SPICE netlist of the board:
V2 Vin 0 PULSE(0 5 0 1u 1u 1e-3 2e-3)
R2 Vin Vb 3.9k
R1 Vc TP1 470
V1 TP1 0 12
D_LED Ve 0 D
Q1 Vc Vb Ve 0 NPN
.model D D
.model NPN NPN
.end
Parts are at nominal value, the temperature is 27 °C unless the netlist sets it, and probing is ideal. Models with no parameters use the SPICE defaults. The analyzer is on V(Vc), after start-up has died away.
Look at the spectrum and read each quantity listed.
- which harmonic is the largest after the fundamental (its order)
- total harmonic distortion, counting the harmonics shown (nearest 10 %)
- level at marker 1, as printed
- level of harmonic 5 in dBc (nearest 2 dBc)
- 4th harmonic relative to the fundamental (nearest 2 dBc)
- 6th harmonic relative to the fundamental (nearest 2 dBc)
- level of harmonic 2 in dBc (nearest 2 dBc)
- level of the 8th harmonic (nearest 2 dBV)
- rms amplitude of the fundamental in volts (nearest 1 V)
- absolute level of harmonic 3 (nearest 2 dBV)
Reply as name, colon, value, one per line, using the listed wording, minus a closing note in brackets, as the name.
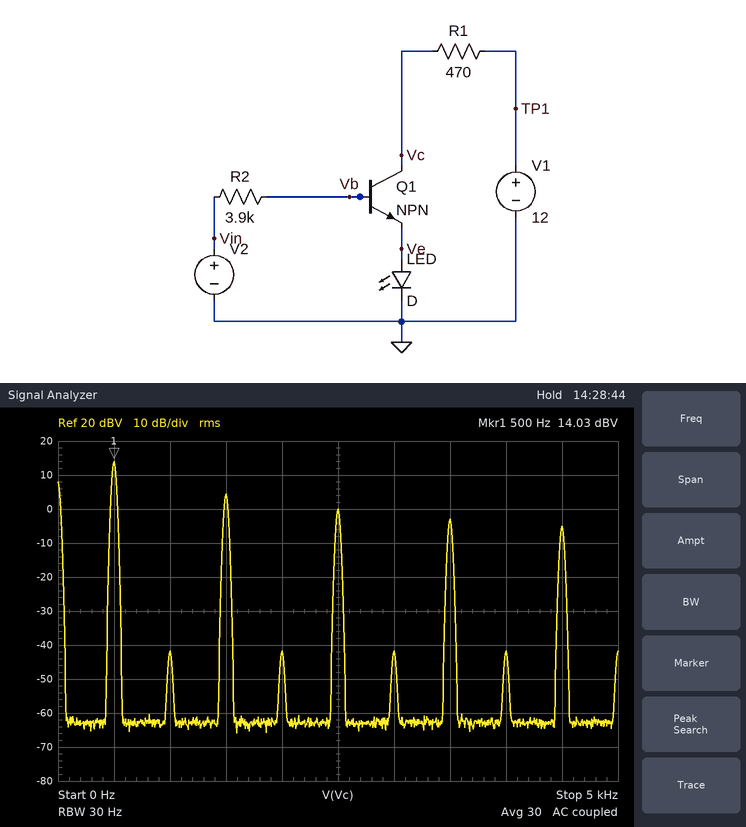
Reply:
which harmonic is the largest after the fundamental: 3
total harmonic distortion, counting the harmonics shown: 40 %
level at marker 1, as printed: 14.03 dBV
level of harmonic 5 in dBc: -14 dBc
4th harmonic relative to the fundamental: -56 dBc
6th harmonic relative to the fundamental: -56 dBc
level of harmonic 2 in dBc: -56 dBc
level of the 8th harmonic: -42 dBV
rms amplitude of the fundamental in volts: 5 V
absolute level of harmonic 3: 4 dBV
